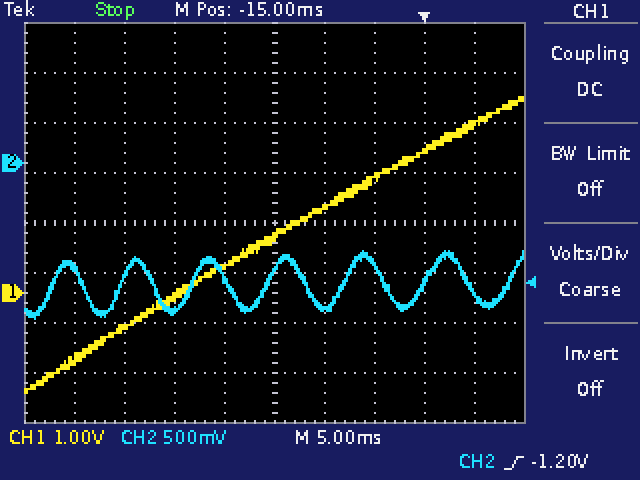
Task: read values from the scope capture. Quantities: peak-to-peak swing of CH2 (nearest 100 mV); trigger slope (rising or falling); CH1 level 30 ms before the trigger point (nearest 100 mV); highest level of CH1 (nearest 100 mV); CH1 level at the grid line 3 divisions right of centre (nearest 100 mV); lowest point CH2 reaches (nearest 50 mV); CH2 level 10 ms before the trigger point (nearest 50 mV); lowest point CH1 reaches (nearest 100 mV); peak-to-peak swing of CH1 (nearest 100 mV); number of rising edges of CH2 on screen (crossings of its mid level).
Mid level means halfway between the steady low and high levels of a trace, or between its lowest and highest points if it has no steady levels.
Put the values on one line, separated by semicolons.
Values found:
700 mV; rising; -700 mV; 3.9 V; 2.9 V; -1.55 V; -1.45 V; -2.0 V; 5.9 V; 7
